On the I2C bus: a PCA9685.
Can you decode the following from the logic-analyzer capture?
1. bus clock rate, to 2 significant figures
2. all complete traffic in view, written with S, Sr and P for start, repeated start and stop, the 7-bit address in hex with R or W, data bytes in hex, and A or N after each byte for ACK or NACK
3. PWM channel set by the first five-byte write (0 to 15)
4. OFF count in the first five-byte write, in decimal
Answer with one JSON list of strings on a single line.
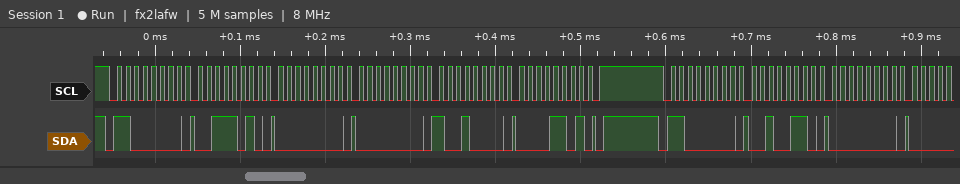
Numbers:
["100 kHz", "S 60W A 3A A 00 A 00 A 90 A 0D A P S 60W A 26 A 00 A", "13", "3472"]
